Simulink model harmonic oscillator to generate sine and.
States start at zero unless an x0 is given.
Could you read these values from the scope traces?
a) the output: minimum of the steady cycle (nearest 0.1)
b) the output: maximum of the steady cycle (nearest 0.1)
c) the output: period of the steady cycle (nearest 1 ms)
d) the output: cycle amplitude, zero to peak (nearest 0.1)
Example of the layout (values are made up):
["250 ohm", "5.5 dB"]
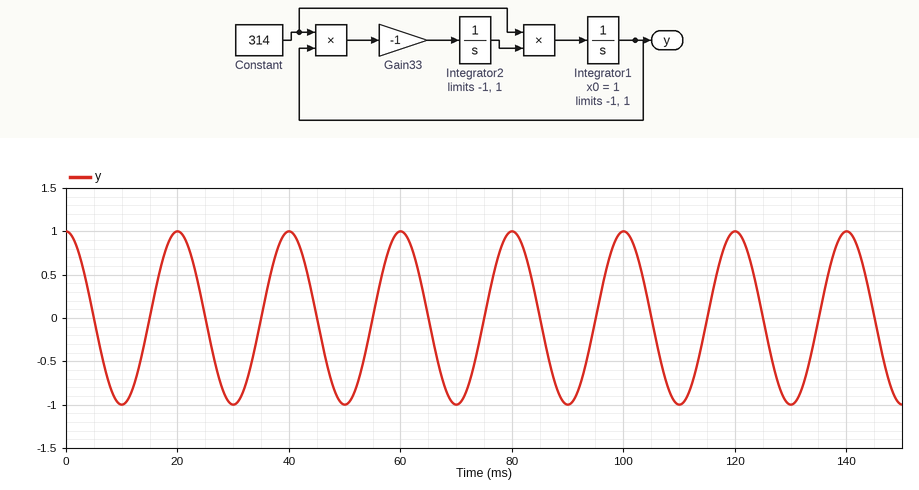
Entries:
["-1.0", "1.0", "20 ms", "1.0"]
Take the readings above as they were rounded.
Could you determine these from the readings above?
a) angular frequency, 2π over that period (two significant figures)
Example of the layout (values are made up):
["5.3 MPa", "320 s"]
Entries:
["0.31 rad/ms"]
